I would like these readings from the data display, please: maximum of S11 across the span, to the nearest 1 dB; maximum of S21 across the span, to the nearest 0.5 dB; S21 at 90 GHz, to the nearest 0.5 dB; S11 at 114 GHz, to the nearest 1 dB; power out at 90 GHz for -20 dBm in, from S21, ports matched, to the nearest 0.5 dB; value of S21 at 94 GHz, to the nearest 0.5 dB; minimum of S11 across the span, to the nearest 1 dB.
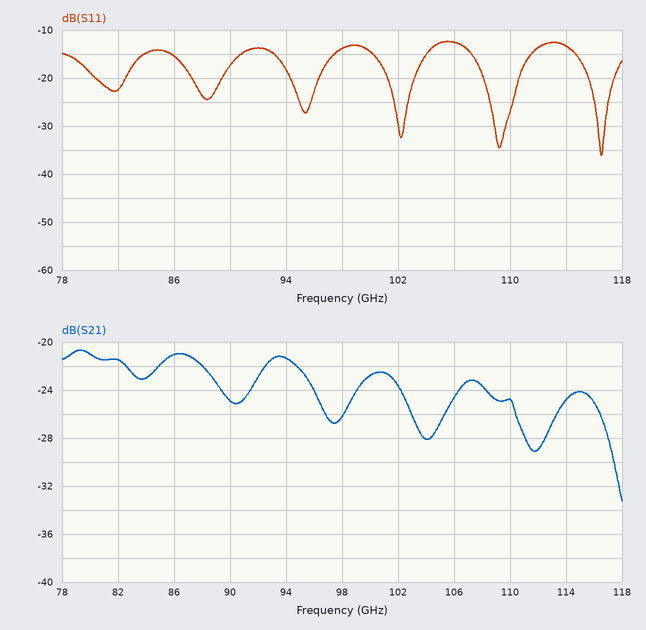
-12 dB
-20.5 dB
-25.0 dB
-13 dB
-45.0 dBm
-21.5 dB
-36 dB
